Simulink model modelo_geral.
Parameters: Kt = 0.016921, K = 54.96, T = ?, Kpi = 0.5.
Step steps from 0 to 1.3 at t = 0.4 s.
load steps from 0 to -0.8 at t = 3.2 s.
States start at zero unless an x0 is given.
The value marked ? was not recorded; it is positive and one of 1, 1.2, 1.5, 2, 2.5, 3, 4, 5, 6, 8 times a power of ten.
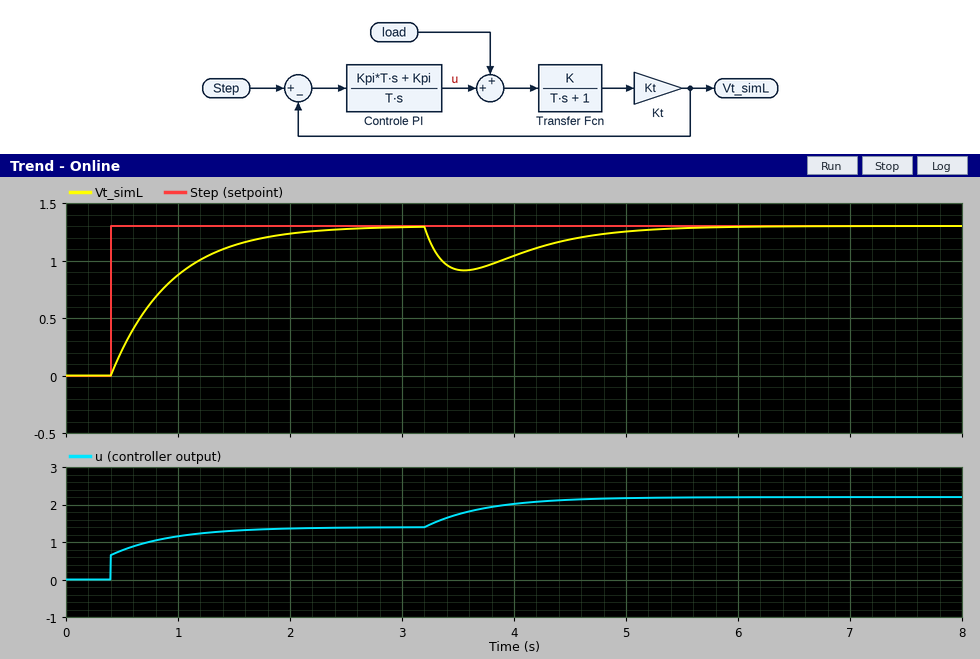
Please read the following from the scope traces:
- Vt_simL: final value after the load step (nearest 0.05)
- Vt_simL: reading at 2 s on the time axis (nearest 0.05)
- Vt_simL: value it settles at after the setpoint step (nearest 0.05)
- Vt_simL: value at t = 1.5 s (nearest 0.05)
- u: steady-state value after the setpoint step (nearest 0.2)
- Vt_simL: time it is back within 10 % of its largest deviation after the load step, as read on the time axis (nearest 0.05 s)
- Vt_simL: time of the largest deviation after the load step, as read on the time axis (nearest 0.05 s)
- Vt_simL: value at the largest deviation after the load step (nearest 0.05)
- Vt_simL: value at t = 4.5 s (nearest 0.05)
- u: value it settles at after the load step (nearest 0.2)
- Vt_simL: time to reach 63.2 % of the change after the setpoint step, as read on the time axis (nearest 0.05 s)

1.30
1.25
1.30
1.15
1.4
5.15 s
3.55 s
0.90
1.20
2.2
0.95 s
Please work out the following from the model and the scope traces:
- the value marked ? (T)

0.25
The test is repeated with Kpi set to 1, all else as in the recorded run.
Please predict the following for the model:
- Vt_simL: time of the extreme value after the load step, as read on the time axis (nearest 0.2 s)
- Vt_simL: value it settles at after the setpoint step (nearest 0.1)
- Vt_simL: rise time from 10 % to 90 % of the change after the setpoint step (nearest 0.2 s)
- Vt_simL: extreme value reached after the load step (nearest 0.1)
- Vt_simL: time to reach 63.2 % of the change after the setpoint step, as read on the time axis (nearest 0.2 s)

3.4 s
1.3
0.6 s
1.0
0.6 s
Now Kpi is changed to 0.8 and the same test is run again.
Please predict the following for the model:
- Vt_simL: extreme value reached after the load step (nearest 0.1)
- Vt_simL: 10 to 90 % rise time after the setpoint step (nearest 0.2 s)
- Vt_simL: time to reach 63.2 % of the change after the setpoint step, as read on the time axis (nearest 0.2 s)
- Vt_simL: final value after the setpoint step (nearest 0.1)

1.0
0.8 s
0.8 s
1.3
